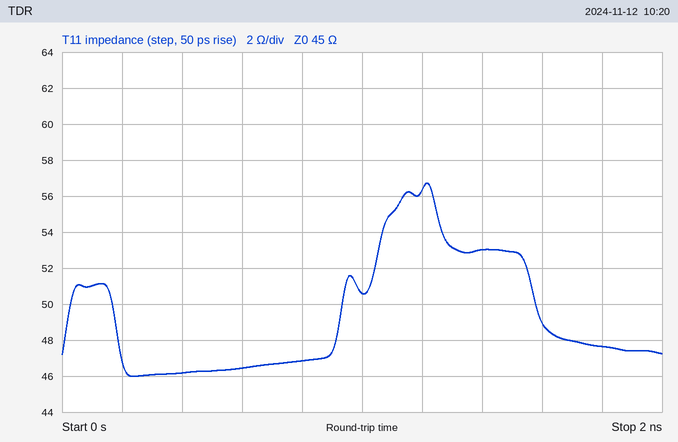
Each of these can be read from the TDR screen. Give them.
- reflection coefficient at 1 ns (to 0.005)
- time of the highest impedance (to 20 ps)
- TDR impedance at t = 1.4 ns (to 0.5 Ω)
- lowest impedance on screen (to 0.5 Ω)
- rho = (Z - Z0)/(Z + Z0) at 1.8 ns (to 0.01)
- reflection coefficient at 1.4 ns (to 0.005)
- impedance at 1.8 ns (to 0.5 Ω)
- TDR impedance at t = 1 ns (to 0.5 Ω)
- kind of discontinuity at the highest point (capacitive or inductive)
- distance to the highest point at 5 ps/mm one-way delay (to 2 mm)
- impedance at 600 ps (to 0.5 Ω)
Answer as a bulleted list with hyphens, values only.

- +0.060
- 1.22 ns
- 53.0 Ω
- 46.0 Ω
- +0.03
- +0.080
- 47.5 Ω
- 50.5 Ω
- inductive
- 122 mm
- 46.5 Ω
